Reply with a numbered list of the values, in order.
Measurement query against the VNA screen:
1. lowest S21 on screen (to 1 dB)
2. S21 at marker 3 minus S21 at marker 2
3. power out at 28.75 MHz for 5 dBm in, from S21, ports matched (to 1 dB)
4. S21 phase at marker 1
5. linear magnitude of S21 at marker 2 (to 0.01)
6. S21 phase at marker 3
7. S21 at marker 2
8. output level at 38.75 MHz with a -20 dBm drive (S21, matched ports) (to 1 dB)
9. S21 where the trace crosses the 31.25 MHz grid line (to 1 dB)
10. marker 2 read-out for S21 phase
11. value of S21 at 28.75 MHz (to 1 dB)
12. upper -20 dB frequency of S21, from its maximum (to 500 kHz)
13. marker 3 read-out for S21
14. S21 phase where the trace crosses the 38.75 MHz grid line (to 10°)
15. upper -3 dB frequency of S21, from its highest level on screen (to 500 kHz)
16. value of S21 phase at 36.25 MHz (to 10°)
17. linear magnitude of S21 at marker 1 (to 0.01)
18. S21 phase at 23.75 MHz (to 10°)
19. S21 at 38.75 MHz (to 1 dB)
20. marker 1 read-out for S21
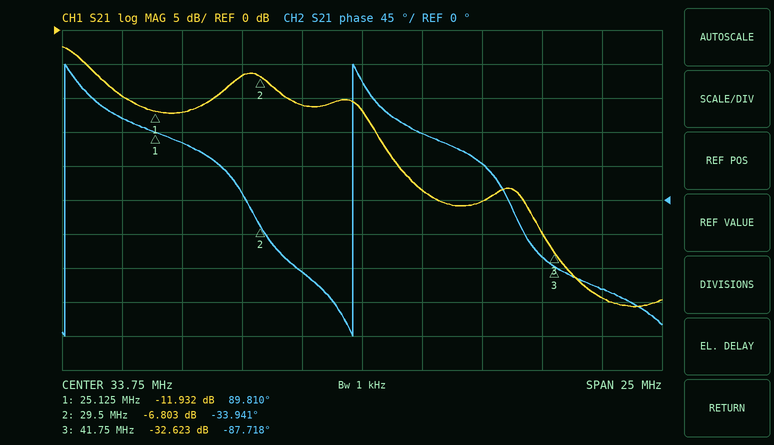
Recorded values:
1. -41 dB
2. -25.820 dB
3. -2 dBm
4. 89.810°
5. 0.46
6. -87.718°
7. -6.803 dB
8. -45 dBm
9. -11 dB
10. -33.941°
11. -7 dB
12. 36.0 MHz
13. -32.623 dB
14. 50°
15. 22.5 MHz
16. 90°
17. 0.25
18. 110°
19. -25 dB
20. -11.932 dB
